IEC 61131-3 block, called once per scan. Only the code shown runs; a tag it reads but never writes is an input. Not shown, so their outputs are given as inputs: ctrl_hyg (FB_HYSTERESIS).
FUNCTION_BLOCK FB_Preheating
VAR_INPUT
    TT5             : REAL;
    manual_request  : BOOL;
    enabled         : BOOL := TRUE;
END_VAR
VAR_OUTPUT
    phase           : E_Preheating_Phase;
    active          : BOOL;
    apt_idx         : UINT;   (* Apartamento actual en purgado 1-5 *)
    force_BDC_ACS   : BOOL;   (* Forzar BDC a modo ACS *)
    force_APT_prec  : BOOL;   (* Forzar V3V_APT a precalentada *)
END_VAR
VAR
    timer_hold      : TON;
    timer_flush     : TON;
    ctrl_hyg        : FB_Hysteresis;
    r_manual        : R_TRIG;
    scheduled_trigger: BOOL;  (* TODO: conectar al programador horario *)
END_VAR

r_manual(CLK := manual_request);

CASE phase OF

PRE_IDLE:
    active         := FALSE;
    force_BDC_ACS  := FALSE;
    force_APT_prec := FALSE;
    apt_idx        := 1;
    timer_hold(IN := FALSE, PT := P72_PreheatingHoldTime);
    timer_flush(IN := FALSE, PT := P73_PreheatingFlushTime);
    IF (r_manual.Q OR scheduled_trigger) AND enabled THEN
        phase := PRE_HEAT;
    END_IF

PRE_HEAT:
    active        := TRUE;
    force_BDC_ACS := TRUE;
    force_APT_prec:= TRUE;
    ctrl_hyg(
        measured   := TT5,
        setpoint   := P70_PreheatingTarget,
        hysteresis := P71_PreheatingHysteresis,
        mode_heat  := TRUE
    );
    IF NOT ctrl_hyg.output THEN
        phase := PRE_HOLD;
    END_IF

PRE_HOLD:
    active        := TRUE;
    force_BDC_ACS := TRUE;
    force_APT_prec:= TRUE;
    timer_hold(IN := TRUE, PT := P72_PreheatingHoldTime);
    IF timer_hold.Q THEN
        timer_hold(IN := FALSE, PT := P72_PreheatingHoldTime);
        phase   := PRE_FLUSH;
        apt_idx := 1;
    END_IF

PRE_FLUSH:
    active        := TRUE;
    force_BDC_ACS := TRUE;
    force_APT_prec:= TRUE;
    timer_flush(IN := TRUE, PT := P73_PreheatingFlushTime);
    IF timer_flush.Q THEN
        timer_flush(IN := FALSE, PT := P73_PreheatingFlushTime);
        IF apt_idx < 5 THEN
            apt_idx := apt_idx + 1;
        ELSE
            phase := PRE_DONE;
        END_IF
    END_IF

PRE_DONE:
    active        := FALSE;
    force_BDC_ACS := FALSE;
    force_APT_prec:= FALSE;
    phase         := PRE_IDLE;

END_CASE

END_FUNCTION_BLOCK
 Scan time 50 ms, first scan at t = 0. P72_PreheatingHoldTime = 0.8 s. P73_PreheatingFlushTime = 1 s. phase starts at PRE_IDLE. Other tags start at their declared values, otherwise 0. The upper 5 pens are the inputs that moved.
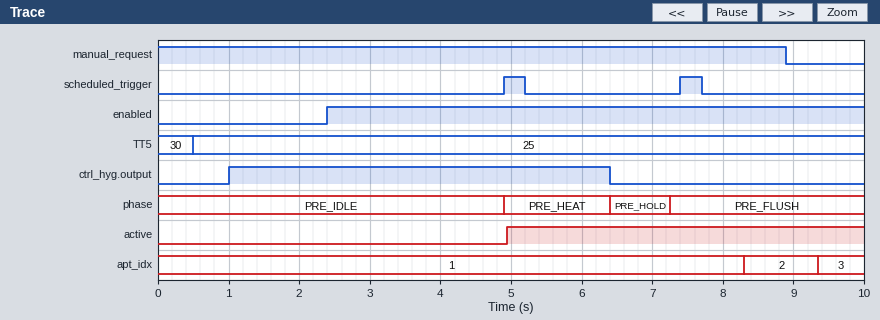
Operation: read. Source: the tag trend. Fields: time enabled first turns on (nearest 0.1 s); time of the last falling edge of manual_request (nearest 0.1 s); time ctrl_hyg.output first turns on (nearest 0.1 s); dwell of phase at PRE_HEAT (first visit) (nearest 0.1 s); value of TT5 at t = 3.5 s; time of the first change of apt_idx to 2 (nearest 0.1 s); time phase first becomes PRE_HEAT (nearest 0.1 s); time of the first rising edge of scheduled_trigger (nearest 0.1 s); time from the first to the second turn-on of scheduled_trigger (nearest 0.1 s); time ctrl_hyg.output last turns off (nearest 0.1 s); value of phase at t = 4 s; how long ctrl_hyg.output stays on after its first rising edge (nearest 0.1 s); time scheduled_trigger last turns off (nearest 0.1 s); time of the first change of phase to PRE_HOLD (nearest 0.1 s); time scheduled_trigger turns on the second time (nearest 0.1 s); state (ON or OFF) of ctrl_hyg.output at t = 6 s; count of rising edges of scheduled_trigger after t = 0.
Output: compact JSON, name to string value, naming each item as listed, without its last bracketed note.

{"time enabled first turns on": "2.4 s", "time of the last falling edge of manual_request": "8.9 s", "time ctrl_hyg.output first turns on": "1.0 s", "dwell of phase at PRE_HEAT (first visit)": "1.5 s", "value of TT5 at t = 3.5 s": "25", "time of the first change of apt_idx to 2": "8.3 s", "time phase first becomes PRE_HEAT": "4.9 s", "time of the first rising edge of scheduled_trigger": "4.9 s", "time from the first to the second turn-on of scheduled_trigger": "2.5 s", "time ctrl_hyg.output last turns off": "6.4 s", "value of phase at t = 4 s": "PRE_IDLE", "how long ctrl_hyg.output stays on after its first rising edge": "5.4 s", "time scheduled_trigger last turns off": "7.7 s", "time of the first change of phase to PRE_HOLD": "6.4 s", "time scheduled_trigger turns on the second time": "7.4 s", "state (ON or OFF) of ctrl_hyg.output at t = 6 s": "ON", "count of rising edges of scheduled_trigger after t = 0": "2"}
